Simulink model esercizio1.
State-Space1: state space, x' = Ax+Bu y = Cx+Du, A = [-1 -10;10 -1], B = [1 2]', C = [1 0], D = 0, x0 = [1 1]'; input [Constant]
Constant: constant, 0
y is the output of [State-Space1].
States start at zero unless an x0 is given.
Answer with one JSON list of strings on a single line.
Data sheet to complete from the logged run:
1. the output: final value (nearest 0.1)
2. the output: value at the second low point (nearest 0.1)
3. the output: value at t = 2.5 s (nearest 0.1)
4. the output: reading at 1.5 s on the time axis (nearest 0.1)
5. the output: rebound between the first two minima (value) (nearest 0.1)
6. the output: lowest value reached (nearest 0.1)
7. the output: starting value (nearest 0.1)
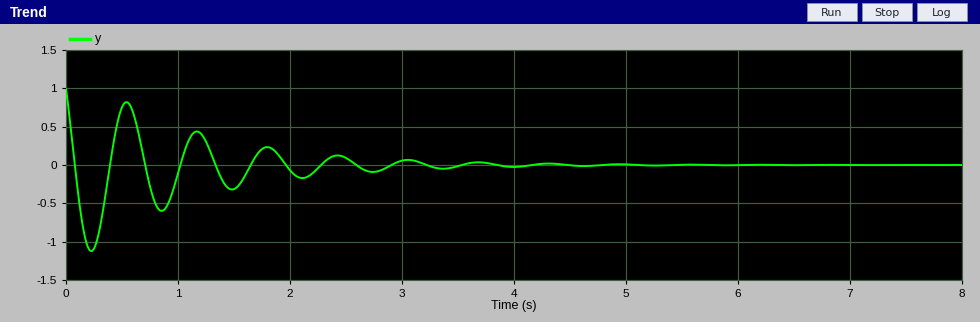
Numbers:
["0.0", "-0.6", "0.1", "-0.3", "0.8", "-1.1", "1.0"]
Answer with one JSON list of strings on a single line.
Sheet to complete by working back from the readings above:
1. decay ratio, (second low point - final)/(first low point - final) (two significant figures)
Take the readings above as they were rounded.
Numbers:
["0.55"]
